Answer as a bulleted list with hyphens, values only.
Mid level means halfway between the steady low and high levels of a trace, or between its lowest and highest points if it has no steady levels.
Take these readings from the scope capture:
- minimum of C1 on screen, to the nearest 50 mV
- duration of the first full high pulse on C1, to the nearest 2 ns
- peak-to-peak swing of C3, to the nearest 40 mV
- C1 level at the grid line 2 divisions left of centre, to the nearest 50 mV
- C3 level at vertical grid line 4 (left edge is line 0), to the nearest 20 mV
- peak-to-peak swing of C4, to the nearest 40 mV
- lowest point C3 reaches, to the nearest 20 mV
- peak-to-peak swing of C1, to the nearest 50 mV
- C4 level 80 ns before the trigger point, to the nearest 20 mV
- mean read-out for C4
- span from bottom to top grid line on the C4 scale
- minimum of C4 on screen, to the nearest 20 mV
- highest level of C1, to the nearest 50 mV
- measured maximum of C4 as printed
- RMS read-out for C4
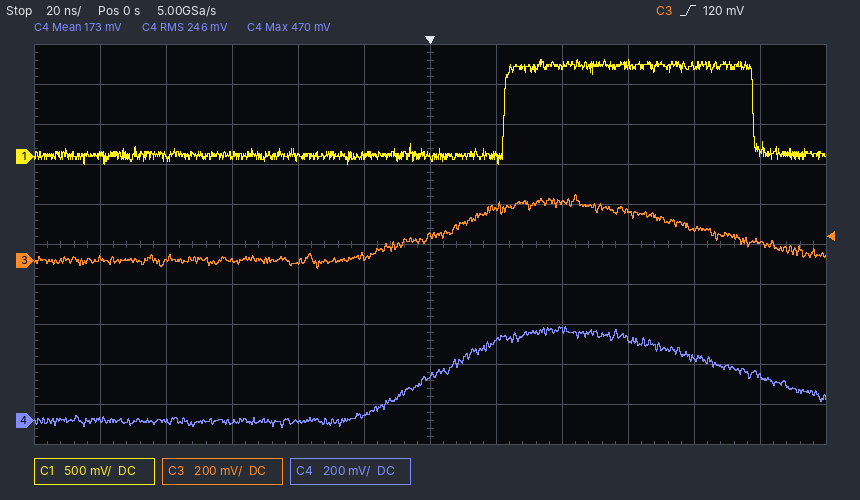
- -100 mV
- 76 ns
- 360 mV
- 0 mV
- 0 mV
- 520 mV
- -40 mV
- 1.30 V
- 0 mV
- 173 mV
- 2 V
- -40 mV
- 1.20 V
- 470 mV
- 246 mV
